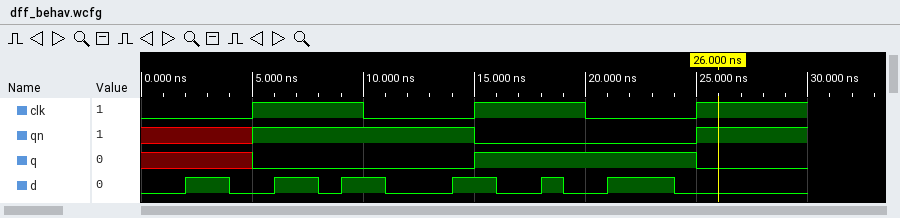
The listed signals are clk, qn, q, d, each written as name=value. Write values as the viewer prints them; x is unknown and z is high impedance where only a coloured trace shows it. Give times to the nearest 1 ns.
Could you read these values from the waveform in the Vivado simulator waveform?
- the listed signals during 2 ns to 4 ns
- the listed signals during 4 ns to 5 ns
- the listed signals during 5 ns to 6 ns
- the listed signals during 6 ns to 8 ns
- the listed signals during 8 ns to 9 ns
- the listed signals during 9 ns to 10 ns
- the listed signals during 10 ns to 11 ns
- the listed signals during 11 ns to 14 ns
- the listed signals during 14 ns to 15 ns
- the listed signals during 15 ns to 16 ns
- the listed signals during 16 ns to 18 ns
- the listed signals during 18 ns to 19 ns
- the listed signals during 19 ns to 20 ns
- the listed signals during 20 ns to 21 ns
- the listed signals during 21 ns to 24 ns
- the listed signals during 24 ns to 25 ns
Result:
clk=0, qn=x, q=x, d=1
clk=0, qn=x, q=x, d=0
clk=1, qn=1, q=0, d=0
clk=1, qn=1, q=0, d=1
clk=1, qn=1, q=0, d=0
clk=1, qn=1, q=0, d=1
clk=0, qn=1, q=0, d=1
clk=0, qn=1, q=0, d=0
clk=0, qn=1, q=0, d=1
clk=1, qn=0, q=1, d=1
clk=1, qn=0, q=1, d=0
clk=1, qn=0, q=1, d=1
clk=1, qn=0, q=1, d=0
clk=0, qn=0, q=1, d=0
clk=0, qn=0, q=1, d=1
clk=0, qn=0, q=1, d=0
